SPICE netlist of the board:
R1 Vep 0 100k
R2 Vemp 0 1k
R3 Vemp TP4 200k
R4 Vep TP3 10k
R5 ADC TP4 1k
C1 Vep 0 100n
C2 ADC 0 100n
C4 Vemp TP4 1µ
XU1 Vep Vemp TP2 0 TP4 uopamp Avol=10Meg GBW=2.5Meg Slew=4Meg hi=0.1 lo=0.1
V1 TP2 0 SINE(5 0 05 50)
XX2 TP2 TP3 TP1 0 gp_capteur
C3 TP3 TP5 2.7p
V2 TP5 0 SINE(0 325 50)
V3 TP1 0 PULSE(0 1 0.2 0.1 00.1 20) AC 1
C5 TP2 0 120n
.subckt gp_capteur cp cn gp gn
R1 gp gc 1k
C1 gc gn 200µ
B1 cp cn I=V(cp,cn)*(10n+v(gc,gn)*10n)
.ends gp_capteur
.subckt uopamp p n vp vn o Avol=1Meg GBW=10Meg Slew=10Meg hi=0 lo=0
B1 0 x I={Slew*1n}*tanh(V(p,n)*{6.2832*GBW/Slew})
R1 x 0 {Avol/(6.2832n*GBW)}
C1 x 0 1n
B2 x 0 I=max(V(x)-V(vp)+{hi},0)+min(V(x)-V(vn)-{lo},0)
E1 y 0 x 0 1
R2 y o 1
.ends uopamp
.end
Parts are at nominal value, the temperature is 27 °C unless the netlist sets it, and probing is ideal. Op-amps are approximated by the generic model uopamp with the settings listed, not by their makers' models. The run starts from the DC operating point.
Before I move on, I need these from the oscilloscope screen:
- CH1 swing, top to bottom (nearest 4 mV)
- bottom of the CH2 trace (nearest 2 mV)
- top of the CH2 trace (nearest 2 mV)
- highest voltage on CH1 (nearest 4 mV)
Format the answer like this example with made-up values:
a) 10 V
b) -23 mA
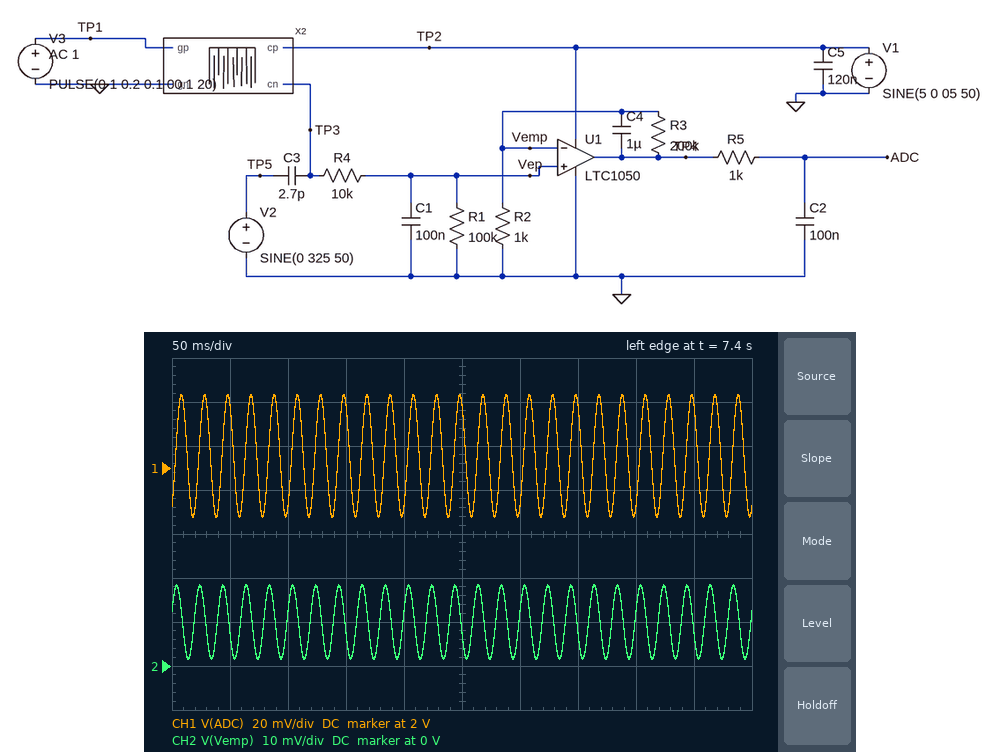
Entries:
a) 56 mV
b) 2 mV
c) 18 mV
d) 2.032 V
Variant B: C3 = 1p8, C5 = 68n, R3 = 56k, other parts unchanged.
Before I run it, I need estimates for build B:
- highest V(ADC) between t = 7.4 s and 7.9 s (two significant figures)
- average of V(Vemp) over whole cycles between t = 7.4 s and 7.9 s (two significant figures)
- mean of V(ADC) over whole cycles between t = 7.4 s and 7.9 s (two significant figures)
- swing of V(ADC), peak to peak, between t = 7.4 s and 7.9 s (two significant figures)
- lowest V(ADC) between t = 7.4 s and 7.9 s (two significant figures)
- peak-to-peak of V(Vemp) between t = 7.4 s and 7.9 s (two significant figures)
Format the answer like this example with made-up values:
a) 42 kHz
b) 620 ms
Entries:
a) 590 mV
b) 10 mV
c) 570 mV
d) 38 mV
e) 550 mV
f) 11 mV
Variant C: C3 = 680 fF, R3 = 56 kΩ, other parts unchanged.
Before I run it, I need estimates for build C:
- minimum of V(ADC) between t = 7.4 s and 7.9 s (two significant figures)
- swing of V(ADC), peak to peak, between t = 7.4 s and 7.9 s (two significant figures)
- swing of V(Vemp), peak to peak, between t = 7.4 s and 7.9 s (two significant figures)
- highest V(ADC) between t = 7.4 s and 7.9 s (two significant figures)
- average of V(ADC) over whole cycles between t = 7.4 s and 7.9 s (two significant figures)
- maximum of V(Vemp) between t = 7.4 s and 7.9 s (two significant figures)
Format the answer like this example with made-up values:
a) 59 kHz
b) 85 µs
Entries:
a) 560 mV
b) 14 mV
c) 4.2 mV
d) 580 mV
e) 570 mV
f) 12 mV
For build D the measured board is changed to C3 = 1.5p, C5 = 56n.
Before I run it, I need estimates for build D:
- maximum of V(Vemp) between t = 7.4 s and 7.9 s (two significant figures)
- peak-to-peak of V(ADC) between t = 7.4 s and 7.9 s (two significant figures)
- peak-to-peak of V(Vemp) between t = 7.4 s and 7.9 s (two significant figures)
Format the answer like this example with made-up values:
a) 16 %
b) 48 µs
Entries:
a) 15 mV
b) 31 mV
c) 9.3 mV
